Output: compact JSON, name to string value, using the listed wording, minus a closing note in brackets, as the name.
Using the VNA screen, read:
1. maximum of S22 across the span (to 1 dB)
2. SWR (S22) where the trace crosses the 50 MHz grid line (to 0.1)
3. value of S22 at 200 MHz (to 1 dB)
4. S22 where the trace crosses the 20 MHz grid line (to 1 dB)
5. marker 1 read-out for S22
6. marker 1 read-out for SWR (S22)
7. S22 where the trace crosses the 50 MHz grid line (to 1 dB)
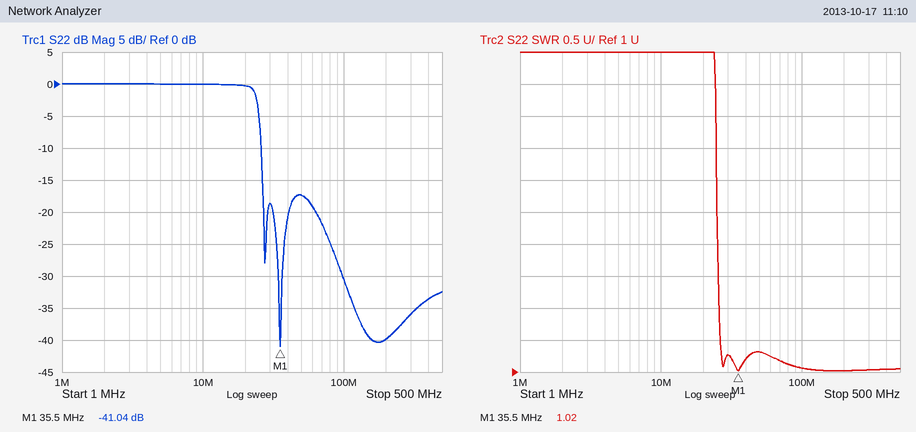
{"maximum of S22 across the span": "0 dB", "SWR (S22) where the trace crosses the 50 MHz grid line": "1.3", "value of S22 at 200 MHz": "-40 dB", "S22 where the trace crosses the 20 MHz grid line": "0 dB", "marker 1 read-out for S22": "-41.04 dB", "marker 1 read-out for SWR": "1.02", "S22 where the trace crosses the 50 MHz grid line": "-17 dB"}
